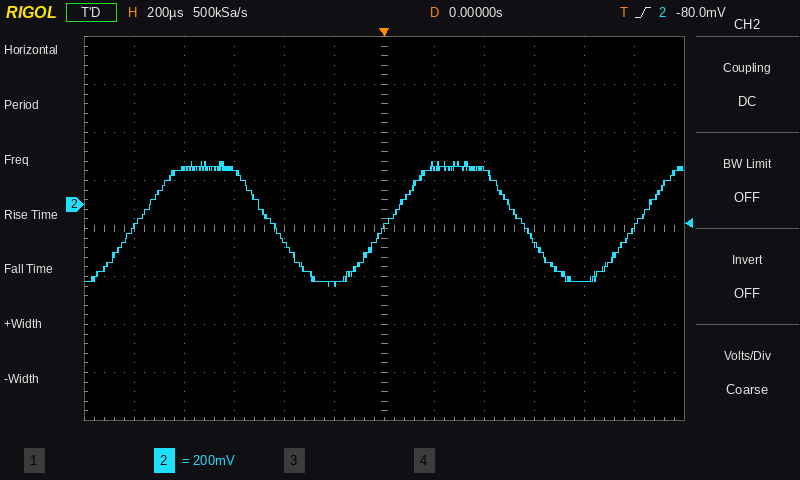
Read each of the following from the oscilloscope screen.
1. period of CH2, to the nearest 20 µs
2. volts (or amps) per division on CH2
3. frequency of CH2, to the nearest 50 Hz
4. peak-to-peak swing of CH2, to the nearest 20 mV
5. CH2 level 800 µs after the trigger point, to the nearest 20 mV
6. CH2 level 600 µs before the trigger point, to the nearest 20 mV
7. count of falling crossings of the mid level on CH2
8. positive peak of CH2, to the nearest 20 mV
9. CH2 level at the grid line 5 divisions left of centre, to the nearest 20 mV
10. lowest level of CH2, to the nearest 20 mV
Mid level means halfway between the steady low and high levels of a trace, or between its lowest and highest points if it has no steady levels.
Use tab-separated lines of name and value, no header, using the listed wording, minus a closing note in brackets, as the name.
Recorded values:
period of CH2, to the nearest 20 µs	1.00 ms
volts (or amps) per division on CH2	200 mV
frequency of CH2, to the nearest 50 Hz	1.00 kHz
peak-to-peak swing of CH2, to the nearest 20 mV	520 mV
CH2 level 800 µs after the trigger point, to the nearest 20 mV	-320 mV
CH2 level 600 µs before the trigger point, to the nearest 20 mV	140 mV
count of falling crossings of the mid level on CH2	2
positive peak of CH2, to the nearest 20 mV	180 mV
CH2 level at the grid line 5 divisions left of centre, to the nearest 20 mV	-100 mV
lowest level of CH2, to the nearest 20 mV	-340 mV
